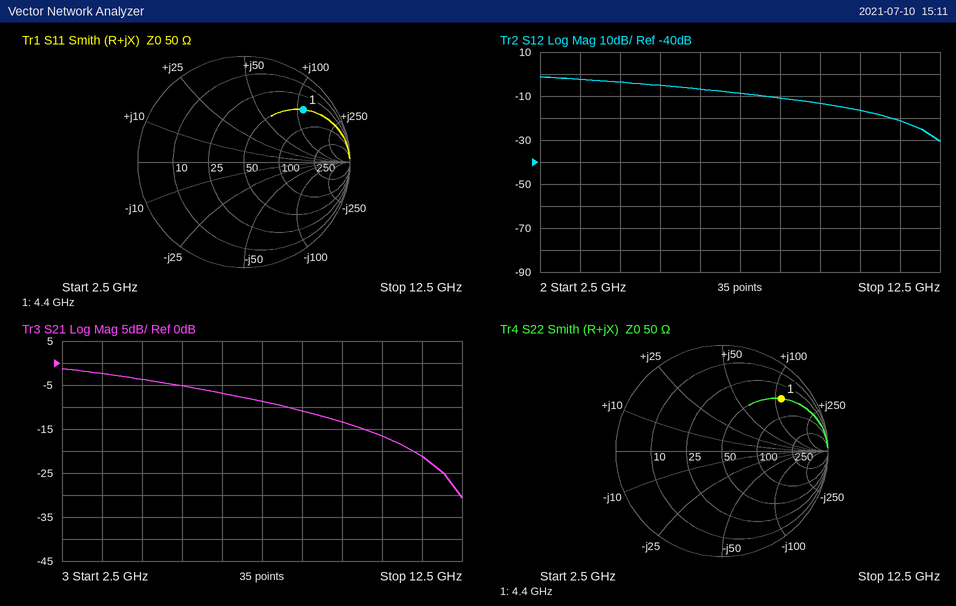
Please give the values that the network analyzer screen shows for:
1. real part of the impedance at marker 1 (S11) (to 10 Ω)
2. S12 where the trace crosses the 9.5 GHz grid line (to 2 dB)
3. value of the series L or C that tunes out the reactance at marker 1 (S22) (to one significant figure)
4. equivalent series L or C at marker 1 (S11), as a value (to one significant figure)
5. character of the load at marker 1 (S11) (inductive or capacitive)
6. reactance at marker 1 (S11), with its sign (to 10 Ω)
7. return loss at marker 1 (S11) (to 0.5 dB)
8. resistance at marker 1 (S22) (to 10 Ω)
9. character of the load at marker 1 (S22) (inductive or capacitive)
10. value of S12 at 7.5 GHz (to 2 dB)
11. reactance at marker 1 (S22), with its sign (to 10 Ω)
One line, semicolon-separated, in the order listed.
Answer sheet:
50 Ω; -14 dB; 300 fF; 4 nH; inductive; +110 Ω; 2.5 dB; 50 Ω; inductive; -8 dB; +110 Ω
